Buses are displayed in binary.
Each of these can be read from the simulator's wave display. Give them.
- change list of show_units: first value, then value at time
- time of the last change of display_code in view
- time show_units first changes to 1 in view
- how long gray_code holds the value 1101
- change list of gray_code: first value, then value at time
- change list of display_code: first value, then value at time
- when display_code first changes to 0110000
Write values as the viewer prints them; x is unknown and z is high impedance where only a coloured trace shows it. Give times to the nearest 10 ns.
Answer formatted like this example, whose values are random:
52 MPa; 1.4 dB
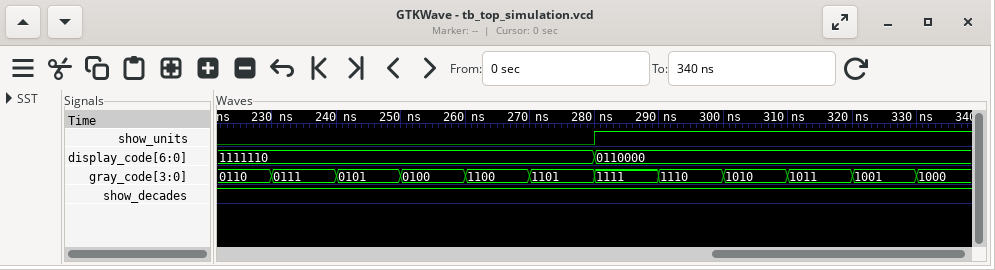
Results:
0, 1 at 280 ns; 280 ns; 280 ns; 10 ns; 0110, 0111 at 230 ns, 0101 at 240 ns, 0100 at 250 ns, 1100 at 260 ns, 1101 at 270 ns, 1111 at 280 ns, 1110 at 290 ns, 1010 at 300 ns, 1011 at 310 ns, 1001 at 320 ns, 1000 at 330 ns; 1111110, 0110000 at 280 ns; 280 ns
